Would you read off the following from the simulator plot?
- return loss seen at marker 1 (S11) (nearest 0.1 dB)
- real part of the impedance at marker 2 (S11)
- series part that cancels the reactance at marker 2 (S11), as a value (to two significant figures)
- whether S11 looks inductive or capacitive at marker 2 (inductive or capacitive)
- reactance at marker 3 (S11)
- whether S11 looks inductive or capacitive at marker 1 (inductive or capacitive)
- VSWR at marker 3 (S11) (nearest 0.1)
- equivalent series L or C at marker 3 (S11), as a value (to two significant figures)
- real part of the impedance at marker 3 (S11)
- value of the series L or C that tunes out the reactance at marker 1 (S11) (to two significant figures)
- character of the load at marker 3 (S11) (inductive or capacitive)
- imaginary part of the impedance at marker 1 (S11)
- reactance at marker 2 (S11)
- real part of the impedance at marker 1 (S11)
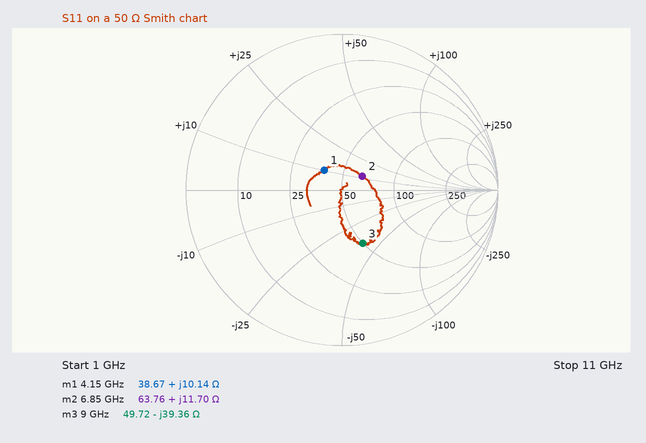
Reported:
15.4 dB
63.76 Ω
2.0 pF
inductive
-39.36 Ω
inductive
2.2
450 fF
49.72 Ω
3.8 pF
capacitive
+10.14 Ω
+11.70 Ω
38.67 Ω
